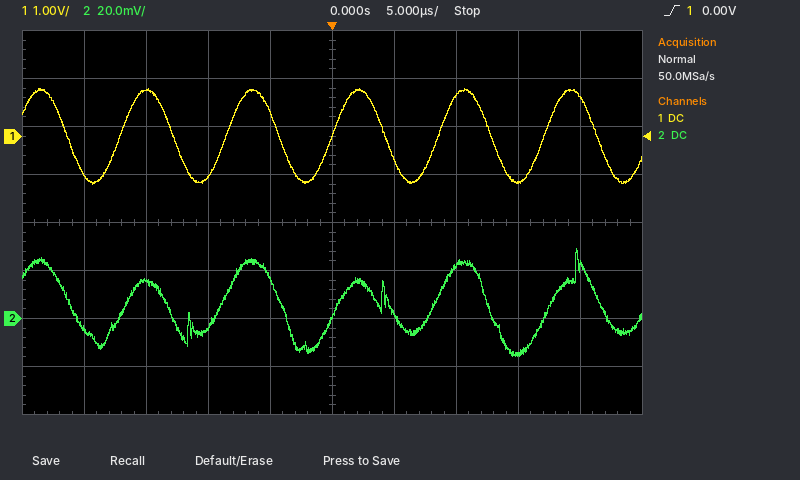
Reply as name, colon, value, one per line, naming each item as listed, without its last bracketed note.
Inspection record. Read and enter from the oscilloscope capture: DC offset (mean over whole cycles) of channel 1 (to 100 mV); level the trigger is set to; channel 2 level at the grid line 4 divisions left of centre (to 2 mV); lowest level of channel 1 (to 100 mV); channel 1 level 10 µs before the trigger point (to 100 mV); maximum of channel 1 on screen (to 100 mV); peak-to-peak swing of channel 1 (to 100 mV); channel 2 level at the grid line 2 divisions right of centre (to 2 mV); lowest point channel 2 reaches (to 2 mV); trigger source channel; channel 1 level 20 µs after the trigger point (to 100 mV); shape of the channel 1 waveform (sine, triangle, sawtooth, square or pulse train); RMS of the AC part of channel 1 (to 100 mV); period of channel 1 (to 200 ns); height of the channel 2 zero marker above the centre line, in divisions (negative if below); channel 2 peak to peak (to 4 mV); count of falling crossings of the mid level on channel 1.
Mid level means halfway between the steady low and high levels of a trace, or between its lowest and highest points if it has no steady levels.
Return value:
DC offset (mean over whole cycles) of channel 1: 0.0 V
level the trigger is set to: 0.00 V
channel 2 level at the grid line 4 divisions left of centre: -4 mV
lowest level of channel 1: -1.0 V
channel 1 level 10 µs before the trigger point: -800 mV
maximum of channel 1 on screen: 1.0 V
peak-to-peak swing of channel 1: 2.0 V
channel 2 level at the grid line 2 divisions right of centre: 22 mV
lowest point channel 2 reaches: -16 mV
trigger source channel: channel 1
channel 1 level 20 µs after the trigger point: 800 mV
shape of the channel 1 waveform: sine
RMS of the AC part of channel 1: 700 mV
period of channel 1: 8.6 µs
height of the channel 2 zero marker above the centre line, in divisions: -2.0 div
channel 2 peak to peak: 44 mV
count of falling crossings of the mid level on channel 1: 6
